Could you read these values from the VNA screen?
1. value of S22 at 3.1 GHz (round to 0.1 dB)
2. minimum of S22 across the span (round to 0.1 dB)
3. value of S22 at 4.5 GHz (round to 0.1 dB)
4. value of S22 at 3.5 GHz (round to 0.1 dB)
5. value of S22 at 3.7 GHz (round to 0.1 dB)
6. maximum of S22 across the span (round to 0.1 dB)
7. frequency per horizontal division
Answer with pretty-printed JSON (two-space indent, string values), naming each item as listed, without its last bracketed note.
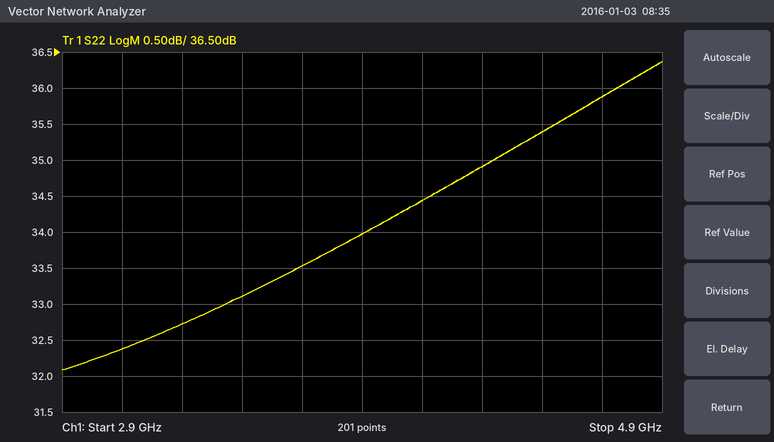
{
  "value of S22 at 3.1 GHz": "32.4 dB",
  "minimum of S22 across the span": "32.1 dB",
  "value of S22 at 4.5 GHz": "35.4 dB",
  "value of S22 at 3.5 GHz": "33.1 dB",
  "value of S22 at 3.7 GHz": "33.5 dB",
  "maximum of S22 across the span": "36.4 dB",
  "frequency per horizontal division": "200 MHz"
}
